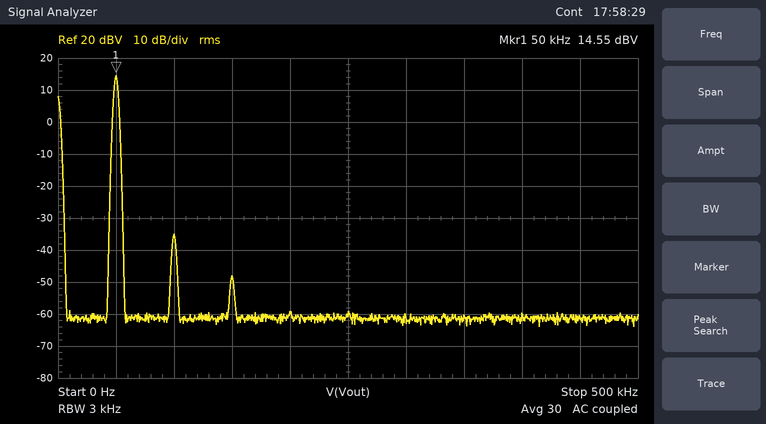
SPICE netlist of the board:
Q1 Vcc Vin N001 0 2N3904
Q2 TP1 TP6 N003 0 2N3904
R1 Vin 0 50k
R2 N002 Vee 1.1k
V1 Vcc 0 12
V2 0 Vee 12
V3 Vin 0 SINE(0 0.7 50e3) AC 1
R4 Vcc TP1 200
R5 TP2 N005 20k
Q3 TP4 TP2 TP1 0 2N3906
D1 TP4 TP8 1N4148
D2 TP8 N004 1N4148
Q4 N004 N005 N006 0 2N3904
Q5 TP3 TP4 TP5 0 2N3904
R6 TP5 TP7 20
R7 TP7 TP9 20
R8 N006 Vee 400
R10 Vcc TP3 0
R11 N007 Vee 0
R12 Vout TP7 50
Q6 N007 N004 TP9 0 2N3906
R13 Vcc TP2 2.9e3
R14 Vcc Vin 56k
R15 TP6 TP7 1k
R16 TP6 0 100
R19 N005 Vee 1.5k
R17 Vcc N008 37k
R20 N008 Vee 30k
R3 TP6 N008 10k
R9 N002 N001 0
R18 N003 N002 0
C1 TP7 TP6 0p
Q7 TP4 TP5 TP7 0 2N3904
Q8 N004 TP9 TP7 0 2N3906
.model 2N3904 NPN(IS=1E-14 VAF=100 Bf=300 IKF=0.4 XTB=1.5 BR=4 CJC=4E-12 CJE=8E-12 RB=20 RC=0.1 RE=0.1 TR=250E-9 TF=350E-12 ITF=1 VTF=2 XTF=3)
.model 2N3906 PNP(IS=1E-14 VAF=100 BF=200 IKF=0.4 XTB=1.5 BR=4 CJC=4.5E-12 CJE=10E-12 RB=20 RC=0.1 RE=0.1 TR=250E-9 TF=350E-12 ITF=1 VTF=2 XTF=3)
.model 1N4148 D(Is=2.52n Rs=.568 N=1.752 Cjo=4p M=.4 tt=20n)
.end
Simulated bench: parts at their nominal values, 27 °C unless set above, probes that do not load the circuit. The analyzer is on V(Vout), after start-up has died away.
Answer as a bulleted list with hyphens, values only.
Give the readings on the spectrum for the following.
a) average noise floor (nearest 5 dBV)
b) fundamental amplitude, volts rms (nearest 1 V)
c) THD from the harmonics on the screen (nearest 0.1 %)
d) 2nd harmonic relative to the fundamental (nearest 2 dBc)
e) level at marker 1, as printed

- -60 dBV
- 5 V
- 0.3 %
- -50 dBc
- 14.55 dBV
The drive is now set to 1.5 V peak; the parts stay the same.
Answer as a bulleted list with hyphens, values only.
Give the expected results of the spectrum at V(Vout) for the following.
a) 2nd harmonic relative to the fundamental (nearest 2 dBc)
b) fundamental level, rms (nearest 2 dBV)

- -24 dBc
- 18 dBV
